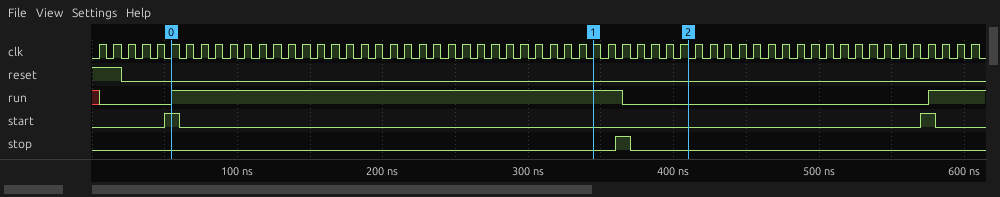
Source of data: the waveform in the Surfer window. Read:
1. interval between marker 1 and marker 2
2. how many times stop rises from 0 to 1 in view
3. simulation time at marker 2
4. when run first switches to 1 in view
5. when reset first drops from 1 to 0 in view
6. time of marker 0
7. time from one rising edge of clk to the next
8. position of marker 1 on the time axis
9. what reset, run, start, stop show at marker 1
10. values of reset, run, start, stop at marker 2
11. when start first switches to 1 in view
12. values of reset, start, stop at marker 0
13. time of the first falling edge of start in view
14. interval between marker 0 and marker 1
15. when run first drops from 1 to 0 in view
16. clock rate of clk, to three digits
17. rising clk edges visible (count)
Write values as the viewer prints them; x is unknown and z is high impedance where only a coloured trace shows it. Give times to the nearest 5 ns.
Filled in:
65 ns
1
410 ns
55 ns
20 ns
55 ns
10 ns
345 ns
reset=0, run=1, start=0, stop=0
reset=0, run=0, start=0, stop=0
50 ns
reset=0, start=1, stop=0
60 ns
290 ns
365 ns
100 MHz
61
